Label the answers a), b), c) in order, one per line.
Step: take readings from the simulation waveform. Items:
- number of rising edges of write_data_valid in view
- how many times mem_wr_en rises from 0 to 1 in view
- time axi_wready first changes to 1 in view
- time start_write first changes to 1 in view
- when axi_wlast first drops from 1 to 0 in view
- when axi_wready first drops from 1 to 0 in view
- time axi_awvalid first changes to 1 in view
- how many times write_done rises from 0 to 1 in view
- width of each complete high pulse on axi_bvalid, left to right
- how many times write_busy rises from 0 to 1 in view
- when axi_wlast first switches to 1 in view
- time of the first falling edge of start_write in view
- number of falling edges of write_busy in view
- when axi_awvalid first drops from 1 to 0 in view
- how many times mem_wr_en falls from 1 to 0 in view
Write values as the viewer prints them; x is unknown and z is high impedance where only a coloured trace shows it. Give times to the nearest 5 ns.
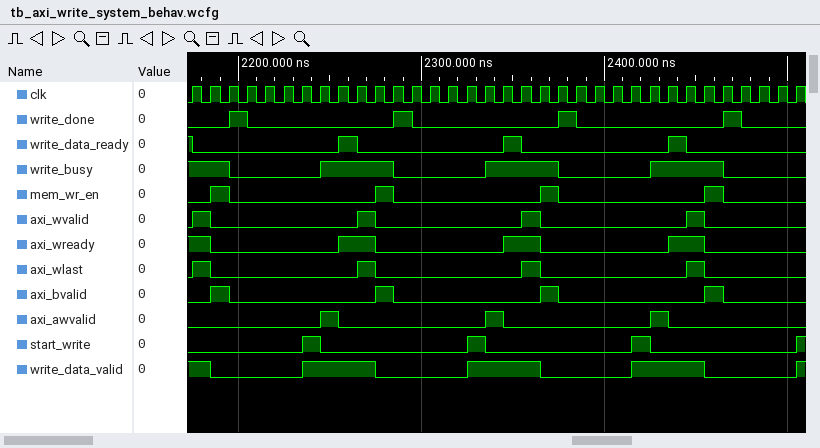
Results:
a) 4
b) 4
c) 2255 ns
d) 2235 ns
e) 2185 ns
f) 2185 ns
g) 2245 ns
h) 4
i) 10 ns, 10 ns, 10 ns, 10 ns
j) 3
k) 2175 ns
l) 2245 ns
m) 4
n) 2255 ns
o) 4
